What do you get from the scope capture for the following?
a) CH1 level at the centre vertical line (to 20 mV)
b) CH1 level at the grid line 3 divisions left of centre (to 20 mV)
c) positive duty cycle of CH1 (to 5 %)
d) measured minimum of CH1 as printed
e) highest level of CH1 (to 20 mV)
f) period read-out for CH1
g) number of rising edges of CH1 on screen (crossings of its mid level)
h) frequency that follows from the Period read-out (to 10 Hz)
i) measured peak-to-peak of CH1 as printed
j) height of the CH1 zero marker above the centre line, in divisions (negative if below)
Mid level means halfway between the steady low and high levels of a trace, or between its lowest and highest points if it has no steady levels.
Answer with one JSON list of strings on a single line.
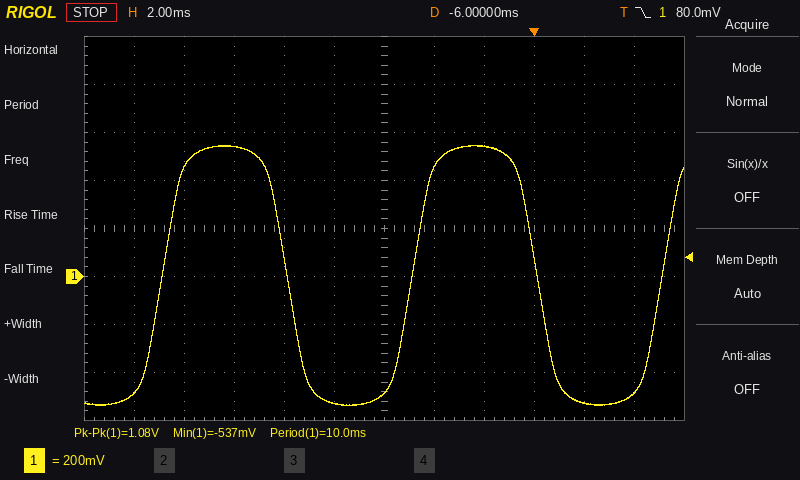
["-480 mV", "540 mV", "50 %", "-537 mV", "540 mV", "10.0 ms", "3", "100 Hz", "1.08 V", "-1.0 div"]
